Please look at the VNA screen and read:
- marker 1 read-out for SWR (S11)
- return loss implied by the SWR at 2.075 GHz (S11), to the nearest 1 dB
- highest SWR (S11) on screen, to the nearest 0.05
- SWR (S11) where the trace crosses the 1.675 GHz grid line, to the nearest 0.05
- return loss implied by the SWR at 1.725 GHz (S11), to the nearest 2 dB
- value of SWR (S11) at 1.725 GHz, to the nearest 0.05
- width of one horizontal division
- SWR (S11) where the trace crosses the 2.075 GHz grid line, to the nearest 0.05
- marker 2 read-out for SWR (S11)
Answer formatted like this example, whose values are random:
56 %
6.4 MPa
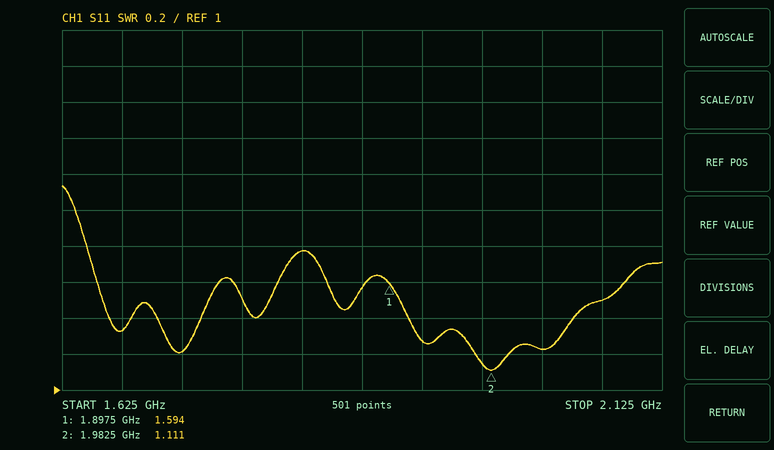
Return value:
1.594
14 dB
2.15
1.35
20 dB
1.20
50 MHz
1.50
1.111
